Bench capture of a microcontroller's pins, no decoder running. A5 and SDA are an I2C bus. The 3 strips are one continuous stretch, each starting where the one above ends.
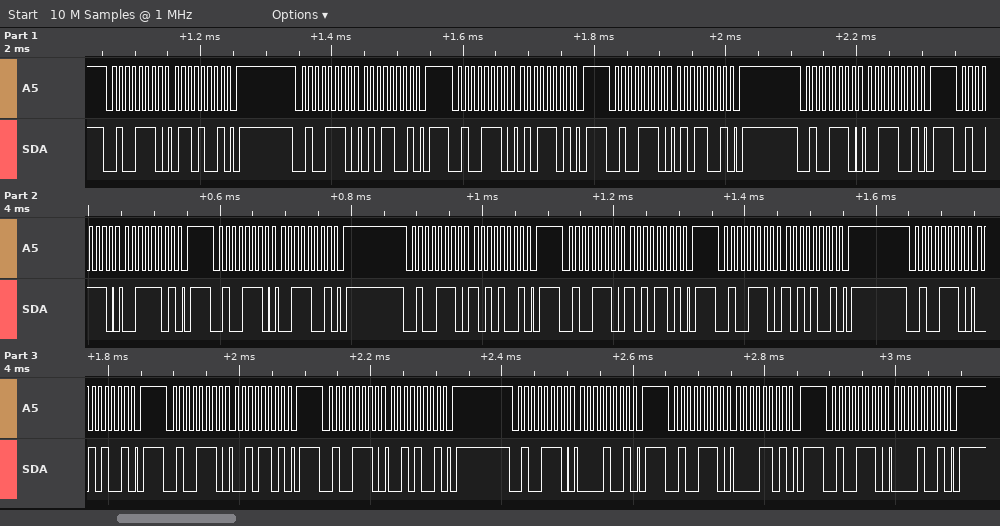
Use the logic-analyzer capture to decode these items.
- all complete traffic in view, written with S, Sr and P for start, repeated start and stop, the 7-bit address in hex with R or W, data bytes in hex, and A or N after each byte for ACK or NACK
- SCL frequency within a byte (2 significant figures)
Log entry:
S 27W A 69 A P S 27W A 59 A P S 27W A 5D A P S 27W A 59 A P S 27W A 39 A P S 27W A 3D A P S 27W A 39 A P S 27W A A9 A P S 27W A AD A P S 27W A A9 A P S 27W A 29 A P S 27W A 2D A P S 27W A 29 A P S 27W A 09 A P S 27W A 0D A P S 27W A 09 A P
100 kHz
